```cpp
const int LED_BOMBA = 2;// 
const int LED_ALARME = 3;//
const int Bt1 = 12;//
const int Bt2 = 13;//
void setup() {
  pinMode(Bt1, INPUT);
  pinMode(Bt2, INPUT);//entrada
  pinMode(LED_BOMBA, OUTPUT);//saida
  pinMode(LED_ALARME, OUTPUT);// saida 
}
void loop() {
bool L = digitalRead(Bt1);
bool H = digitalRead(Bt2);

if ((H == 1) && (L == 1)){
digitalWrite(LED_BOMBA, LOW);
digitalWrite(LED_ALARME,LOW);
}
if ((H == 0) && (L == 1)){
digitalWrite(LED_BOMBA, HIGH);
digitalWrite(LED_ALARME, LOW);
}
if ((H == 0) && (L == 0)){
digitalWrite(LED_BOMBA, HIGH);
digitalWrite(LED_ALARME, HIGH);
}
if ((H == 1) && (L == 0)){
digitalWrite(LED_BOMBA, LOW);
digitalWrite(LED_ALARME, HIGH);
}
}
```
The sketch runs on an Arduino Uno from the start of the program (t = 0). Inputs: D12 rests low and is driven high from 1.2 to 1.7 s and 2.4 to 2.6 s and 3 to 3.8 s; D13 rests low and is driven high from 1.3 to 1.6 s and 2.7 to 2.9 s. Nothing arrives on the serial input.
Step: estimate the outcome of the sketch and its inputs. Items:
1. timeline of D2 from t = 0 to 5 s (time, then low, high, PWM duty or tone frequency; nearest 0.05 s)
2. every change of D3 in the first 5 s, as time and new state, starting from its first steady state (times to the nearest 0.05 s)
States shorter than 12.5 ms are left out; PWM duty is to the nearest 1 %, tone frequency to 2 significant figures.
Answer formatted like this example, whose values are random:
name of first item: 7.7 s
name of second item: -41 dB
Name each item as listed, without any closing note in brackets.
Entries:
timeline of D2 from t = 0 to 5 s: 0 s high; 1.3 s low; 1.6 s high; 2.7 s low; 2.9 s high
every change of D3 in the first 5 s, as time and new state, starting from its first steady state: 0 s high; 1.2 s low; 1.7 s high; 2.4 s low; 2.6 s high; 3 s low; 3.8 s high
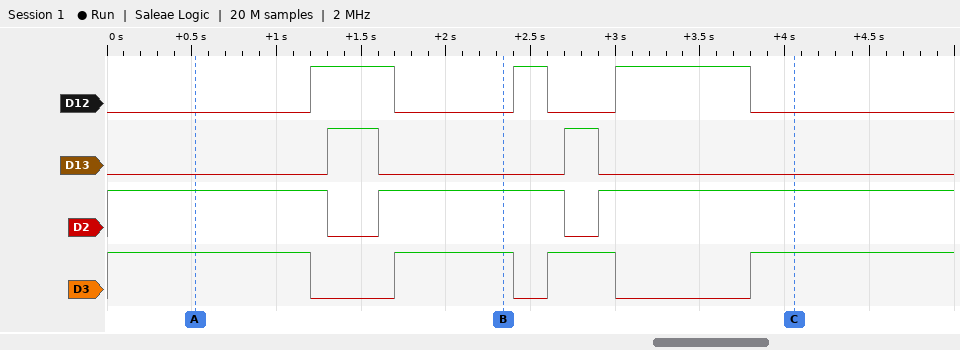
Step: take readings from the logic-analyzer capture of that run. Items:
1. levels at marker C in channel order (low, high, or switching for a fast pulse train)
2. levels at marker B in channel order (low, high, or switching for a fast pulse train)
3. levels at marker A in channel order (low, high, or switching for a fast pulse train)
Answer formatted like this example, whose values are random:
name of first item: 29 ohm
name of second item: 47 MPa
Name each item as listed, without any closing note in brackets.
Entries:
levels at marker C in channel order: D12 low, D13 low, D2 high, D3 high
levels at marker B in channel order: D12 low, D13 low, D2 high, D3 high
levels at marker A in channel order: D12 low, D13 low, D2 high, D3 high
